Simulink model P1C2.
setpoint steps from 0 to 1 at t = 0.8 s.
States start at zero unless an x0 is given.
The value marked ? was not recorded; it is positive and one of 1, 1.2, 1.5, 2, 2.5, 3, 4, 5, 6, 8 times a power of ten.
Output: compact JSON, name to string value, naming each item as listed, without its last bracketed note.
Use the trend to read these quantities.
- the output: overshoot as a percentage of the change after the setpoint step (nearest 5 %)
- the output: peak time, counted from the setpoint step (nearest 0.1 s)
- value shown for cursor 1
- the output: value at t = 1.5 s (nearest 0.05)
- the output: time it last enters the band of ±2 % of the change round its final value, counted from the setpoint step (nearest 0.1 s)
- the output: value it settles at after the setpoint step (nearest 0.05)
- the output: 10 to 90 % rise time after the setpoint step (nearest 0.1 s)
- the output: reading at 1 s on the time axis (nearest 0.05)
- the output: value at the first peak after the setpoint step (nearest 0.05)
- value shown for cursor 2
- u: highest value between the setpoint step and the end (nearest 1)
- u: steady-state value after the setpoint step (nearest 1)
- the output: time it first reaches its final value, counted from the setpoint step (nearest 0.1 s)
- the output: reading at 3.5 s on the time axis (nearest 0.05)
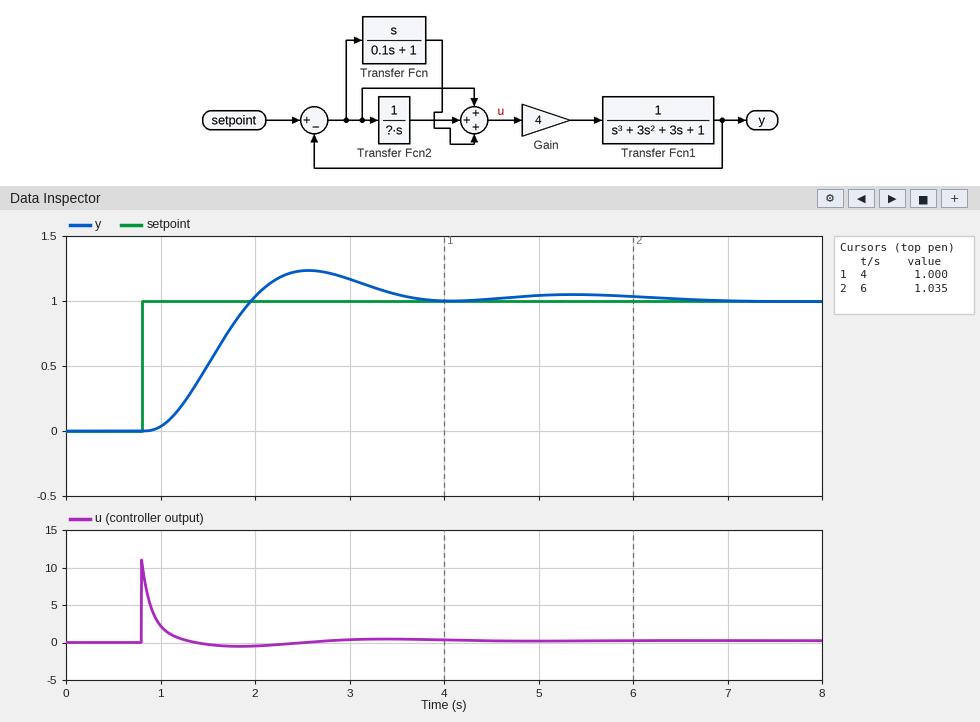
{"the output: overshoot as a percentage of the change after the setpoint step": "25 %", "the output: peak time, counted from the setpoint step": "1.8 s", "value shown for cursor 1": "1.000", "the output: value at t = 1.5 s": "0.50", "the output: time it last enters the band of ±2 % of the change round its final value, counted from the setpoint step": "5.6 s", "the output: value it settles at after the setpoint step": "1.00", "the output: 10 to 90 % rise time after the setpoint step": "0.7 s", "the output: reading at 1 s on the time axis": "0.05", "the output: value at the first peak after the setpoint step": "1.25", "value shown for cursor 2": "1.035", "u: highest value between the setpoint step and the end": "11", "u: steady-state value after the setpoint step": "0", "the output: time it first reaches its final value, counted from the setpoint step": "1.2 s", "the output: reading at 3.5 s on the time axis": "1.05"}
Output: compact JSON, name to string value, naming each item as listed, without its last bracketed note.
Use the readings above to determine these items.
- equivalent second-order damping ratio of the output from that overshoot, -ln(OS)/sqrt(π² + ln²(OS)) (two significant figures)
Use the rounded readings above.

{"equivalent second-order damping ratio of the output from that overshoot, -ln(OS)/sqrt(π² + ln²(OS))": "0.40"}
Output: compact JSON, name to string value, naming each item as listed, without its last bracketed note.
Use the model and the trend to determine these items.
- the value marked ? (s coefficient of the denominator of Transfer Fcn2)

{"the value marked ?": "1.5"}
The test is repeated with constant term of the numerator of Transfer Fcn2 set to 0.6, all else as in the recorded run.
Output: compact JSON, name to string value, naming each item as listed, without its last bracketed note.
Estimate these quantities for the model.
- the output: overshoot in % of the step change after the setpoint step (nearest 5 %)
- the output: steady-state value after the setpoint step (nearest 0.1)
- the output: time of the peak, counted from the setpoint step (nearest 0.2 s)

{"the output: overshoot in % of the step change after the setpoint step": "15 %", "the output: steady-state value after the setpoint step": "1.0", "the output: time of the peak, counted from the setpoint step": "1.6 s"}
